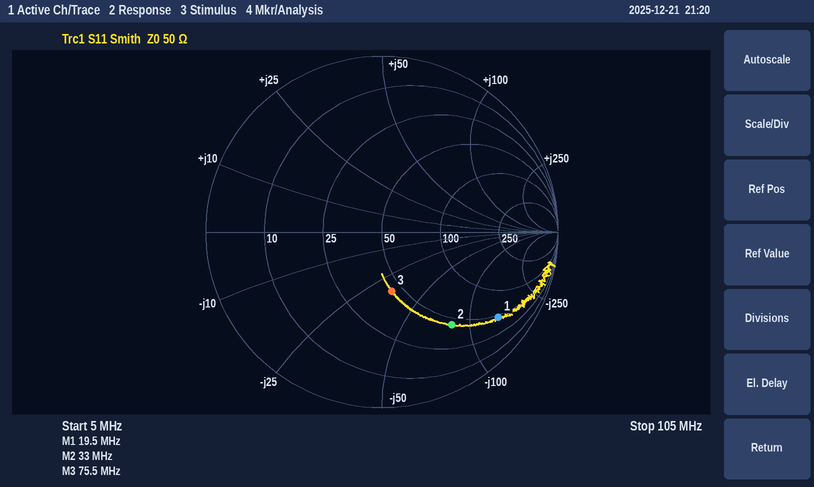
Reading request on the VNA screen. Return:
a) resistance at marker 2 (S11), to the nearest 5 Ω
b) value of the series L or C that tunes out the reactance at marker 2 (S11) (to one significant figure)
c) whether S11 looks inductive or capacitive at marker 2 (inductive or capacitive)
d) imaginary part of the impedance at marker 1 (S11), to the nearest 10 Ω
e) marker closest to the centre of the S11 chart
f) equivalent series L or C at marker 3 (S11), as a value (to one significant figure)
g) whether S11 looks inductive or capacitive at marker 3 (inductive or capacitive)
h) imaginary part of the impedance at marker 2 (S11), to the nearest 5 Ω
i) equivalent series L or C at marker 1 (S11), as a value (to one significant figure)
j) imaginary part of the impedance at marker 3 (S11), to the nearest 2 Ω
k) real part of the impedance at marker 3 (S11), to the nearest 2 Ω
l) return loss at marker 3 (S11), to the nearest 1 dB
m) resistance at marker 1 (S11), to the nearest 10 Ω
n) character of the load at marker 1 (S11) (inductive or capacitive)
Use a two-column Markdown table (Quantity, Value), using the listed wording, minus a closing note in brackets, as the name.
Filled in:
| Quantity | Value |
|---|---|
| resistance at marker 2 (S11), to the nearest 5 Ω | 45 Ω |
| value of the series L or C that tunes out the reactance at marker 2 (S11) | 400 nH |
| whether S11 looks inductive or capacitive at marker 2 | capacitive |
| imaginary part of the impedance at marker 1 (S11), to the nearest 10 Ω | -140 Ω |
| marker closest to the centre of the S11 chart | marker 3 |
| equivalent series L or C at marker 3 (S11), as a value | 60 pF |
| whether S11 looks inductive or capacitive at marker 3 | capacitive |
| imaginary part of the impedance at marker 2 (S11), to the nearest 5 Ω | -80 Ω |
| equivalent series L or C at marker 1 (S11), as a value | 60 pF |
| imaginary part of the impedance at marker 3 (S11), to the nearest 2 Ω | -34 Ω |
| real part of the impedance at marker 3 (S11), to the nearest 2 Ω | 44 Ω |
| return loss at marker 3 (S11), to the nearest 1 dB | 9 dB |
| resistance at marker 1 (S11), to the nearest 10 Ω | 50 Ω |
| character of the load at marker 1 (S11) | capacitive |
